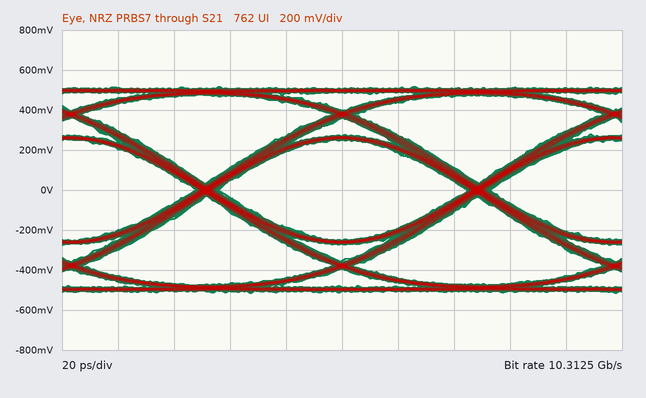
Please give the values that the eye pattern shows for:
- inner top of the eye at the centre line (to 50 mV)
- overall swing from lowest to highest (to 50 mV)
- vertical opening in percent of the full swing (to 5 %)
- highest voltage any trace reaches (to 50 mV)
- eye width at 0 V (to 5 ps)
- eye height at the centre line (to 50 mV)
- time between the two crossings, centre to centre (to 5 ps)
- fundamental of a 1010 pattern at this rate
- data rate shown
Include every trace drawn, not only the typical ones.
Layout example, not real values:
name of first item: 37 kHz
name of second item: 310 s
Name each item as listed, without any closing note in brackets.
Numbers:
inner top of the eye at the centre line: 250 mV
overall swing from lowest to highest: 1.05 V
vertical opening in percent of the full swing: 50 %
highest voltage any trace reaches: 500 mV
eye width at 0 V: 90 ps
eye height at the centre line: 500 mV
time between the two crossings, centre to centre: 95 ps
fundamental of a 1010 pattern at this rate: 5.15625 GHz
data rate shown: 10.3125 Gb/s
